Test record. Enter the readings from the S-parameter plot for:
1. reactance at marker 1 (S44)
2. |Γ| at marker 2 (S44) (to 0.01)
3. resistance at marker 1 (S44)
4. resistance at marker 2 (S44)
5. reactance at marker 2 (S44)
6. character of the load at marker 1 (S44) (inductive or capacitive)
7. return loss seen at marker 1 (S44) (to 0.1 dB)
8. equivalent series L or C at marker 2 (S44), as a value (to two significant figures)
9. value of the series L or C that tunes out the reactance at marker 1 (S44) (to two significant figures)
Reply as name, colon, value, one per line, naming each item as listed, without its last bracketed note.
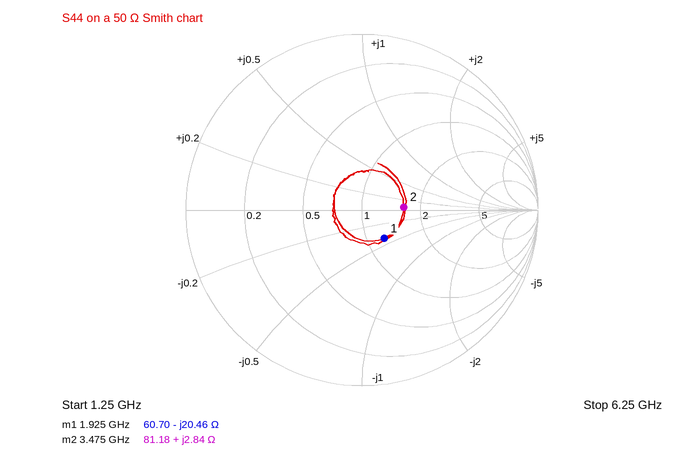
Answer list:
reactance at marker 1: -20.46 Ω
|Γ| at marker 2 (S44): 0.24
resistance at marker 1: 60.70 Ω
resistance at marker 2: 81.18 Ω
reactance at marker 2: +2.84 Ω
character of the load at marker 1 (S44): capacitive
return loss seen at marker 1 (S44): 13.8 dB
equivalent series L or C at marker 2 (S44), as a value: 130 pH
value of the series L or C that tunes out the reactance at marker 1 (S44): 1.7 nH
